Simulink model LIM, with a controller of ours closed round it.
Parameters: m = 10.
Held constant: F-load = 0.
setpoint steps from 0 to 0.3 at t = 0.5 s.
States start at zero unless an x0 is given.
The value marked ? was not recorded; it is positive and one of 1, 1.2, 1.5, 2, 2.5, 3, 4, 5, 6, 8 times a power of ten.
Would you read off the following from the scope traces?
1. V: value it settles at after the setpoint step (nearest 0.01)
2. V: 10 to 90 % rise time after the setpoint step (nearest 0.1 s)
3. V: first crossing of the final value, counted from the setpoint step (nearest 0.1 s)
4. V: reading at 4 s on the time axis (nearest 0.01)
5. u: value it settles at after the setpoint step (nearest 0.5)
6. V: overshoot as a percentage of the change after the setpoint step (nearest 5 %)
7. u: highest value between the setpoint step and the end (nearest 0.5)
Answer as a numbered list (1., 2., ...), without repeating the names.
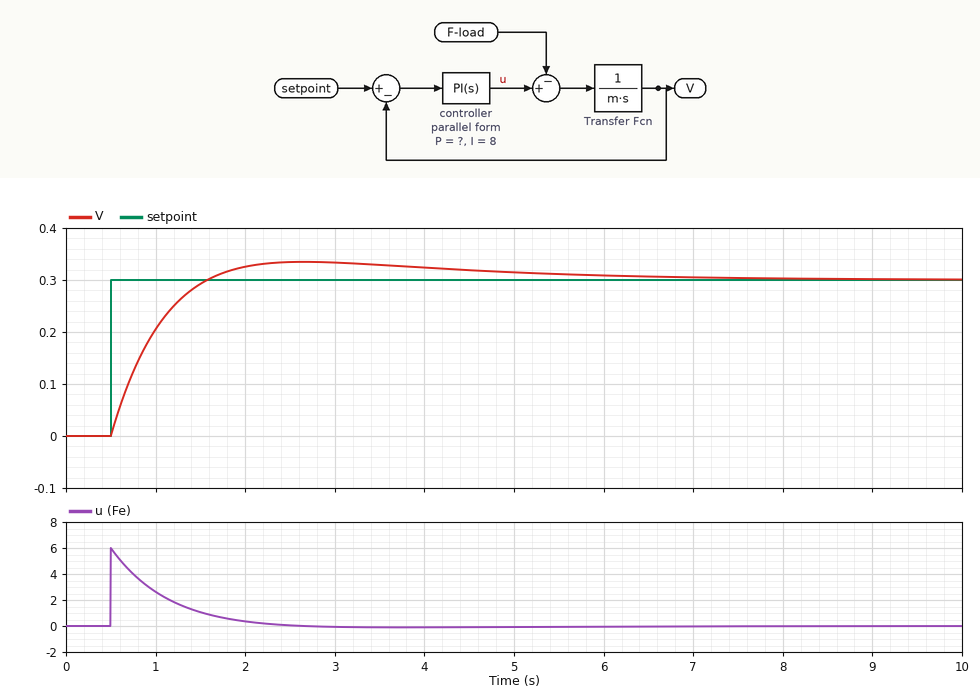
1. 0.30
2. 0.8 s
3. 1.1 s
4. 0.32
5. 0.0
6. 10 %
7. 6.0
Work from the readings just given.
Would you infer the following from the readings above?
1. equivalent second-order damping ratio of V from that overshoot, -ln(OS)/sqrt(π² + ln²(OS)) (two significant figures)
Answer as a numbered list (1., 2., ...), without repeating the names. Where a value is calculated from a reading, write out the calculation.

1. ln(0.1) = -2.303; 2.303 / sqrt(9.870 + 5.302) = 0.59
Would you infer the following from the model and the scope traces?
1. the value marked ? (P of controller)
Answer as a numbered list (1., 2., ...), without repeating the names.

1. 20
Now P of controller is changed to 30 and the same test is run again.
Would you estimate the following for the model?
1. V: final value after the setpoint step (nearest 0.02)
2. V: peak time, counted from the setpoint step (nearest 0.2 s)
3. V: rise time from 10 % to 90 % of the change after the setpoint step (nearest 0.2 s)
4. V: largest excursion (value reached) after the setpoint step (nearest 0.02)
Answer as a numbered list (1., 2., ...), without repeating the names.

1. 0.30
2. 1.8 s
3. 0.6 s
4. 0.32
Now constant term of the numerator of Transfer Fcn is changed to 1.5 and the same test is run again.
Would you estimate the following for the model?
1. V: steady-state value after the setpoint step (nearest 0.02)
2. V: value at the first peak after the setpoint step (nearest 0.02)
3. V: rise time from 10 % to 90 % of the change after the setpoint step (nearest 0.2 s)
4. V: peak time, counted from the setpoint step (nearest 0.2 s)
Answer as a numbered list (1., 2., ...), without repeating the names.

1. 0.30
2. 0.32
3. 0.6 s
4. 1.6 s
